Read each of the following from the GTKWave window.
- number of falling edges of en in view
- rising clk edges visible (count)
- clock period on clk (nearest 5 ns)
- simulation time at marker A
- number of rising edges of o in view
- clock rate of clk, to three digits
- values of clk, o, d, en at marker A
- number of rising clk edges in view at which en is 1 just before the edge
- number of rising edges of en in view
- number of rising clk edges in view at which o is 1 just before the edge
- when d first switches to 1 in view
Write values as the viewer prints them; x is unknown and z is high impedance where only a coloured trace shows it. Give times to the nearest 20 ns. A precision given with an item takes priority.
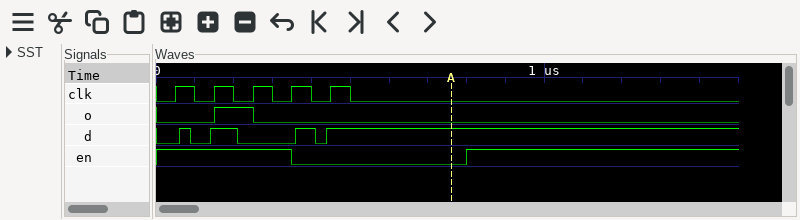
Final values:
1
5
100 ns
760 ns
1
10.0 MHz
clk=0, o=0, d=1, en=0
4
1
1
60 ns
